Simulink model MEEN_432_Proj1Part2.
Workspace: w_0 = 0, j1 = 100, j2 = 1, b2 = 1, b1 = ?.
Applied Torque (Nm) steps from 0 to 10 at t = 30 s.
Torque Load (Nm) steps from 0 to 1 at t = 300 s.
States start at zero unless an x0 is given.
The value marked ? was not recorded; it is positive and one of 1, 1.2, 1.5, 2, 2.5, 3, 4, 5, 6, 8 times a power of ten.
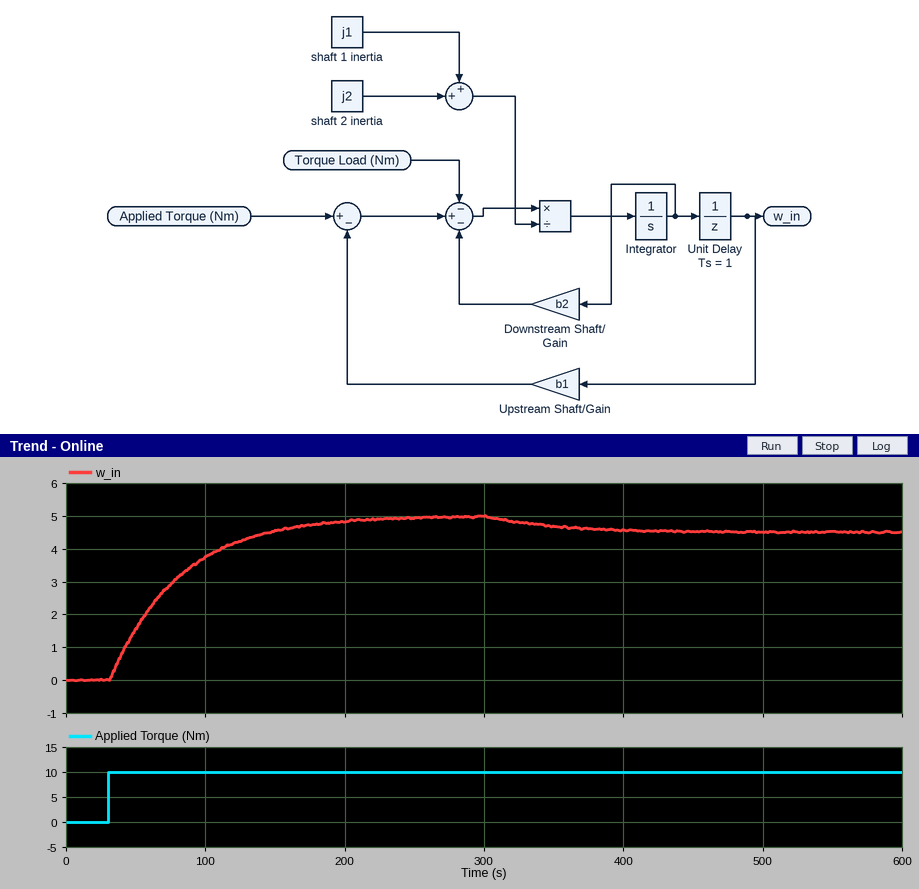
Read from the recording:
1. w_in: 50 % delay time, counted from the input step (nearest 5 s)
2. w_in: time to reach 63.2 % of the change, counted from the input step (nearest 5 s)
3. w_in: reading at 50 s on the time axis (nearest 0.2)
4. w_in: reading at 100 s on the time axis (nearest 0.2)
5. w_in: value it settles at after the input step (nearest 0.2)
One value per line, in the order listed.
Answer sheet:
35 s
50 s
1.6
3.8
5.0
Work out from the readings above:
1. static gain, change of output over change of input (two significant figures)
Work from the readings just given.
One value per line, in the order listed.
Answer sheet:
0.50
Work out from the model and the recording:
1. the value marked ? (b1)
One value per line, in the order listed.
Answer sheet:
1
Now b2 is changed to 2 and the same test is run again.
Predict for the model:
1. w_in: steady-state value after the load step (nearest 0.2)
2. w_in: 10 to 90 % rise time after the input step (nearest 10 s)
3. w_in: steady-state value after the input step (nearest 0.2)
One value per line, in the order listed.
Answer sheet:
3.0
70 s
3.4
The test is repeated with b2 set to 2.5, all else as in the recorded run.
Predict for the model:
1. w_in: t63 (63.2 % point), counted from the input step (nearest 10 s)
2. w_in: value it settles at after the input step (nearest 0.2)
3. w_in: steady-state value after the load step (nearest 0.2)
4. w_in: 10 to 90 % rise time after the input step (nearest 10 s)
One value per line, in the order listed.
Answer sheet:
30 s
2.8
2.6
60 s
